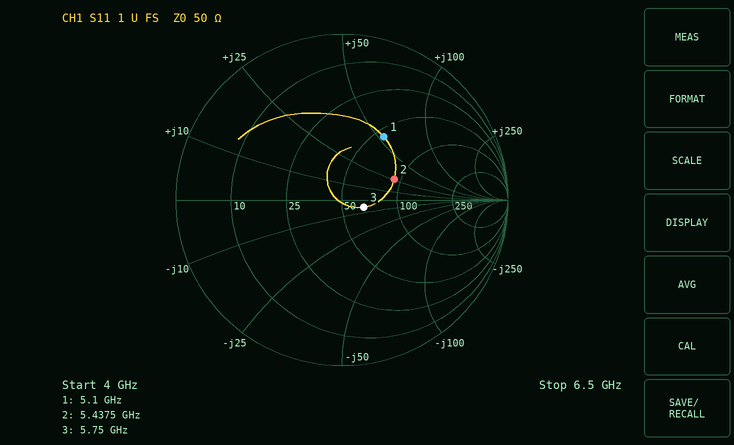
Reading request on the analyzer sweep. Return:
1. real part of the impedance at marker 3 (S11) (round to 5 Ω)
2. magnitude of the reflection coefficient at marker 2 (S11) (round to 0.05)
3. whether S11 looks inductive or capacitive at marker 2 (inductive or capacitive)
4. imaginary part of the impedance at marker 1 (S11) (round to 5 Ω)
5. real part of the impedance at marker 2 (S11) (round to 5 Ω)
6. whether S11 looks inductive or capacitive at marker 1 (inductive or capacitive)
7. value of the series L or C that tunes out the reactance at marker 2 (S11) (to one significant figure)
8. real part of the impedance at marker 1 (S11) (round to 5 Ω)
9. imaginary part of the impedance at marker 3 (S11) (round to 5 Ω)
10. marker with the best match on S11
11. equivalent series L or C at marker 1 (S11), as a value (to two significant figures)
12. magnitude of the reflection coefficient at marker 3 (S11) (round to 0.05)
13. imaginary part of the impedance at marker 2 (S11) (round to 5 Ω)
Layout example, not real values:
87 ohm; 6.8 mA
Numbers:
65 Ω; 0.35; inductive; +55 Ω; 90 Ω; inductive; 1 pF; 55 Ω; -5 Ω; marker 3; 1.7 nH; 0.15; +25 Ω
